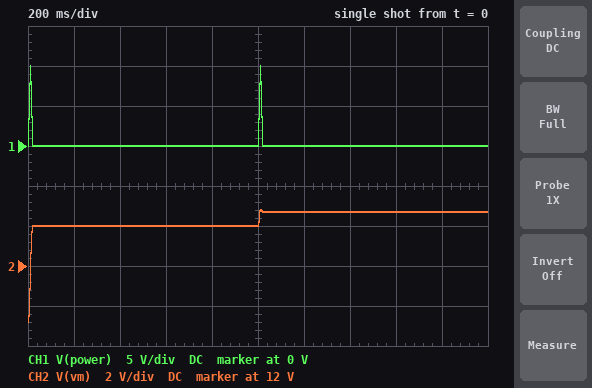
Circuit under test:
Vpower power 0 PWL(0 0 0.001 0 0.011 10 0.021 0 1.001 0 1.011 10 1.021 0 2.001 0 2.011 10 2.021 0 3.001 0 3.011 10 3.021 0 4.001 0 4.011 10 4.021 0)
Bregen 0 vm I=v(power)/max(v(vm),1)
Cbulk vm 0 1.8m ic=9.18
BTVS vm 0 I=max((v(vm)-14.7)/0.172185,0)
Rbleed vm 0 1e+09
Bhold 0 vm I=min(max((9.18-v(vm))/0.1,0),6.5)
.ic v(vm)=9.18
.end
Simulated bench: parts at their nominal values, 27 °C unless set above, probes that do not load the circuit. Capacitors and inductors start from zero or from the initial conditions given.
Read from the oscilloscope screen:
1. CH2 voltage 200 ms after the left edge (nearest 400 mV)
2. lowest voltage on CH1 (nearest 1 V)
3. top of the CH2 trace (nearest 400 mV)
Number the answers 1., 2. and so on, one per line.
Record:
1. 14.0 V
2. 0 V
3. 14.8 V
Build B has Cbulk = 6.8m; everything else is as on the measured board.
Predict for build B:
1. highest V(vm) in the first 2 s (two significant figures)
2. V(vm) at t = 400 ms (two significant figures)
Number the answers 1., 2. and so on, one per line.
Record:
1. 12 V
2. 11 V
